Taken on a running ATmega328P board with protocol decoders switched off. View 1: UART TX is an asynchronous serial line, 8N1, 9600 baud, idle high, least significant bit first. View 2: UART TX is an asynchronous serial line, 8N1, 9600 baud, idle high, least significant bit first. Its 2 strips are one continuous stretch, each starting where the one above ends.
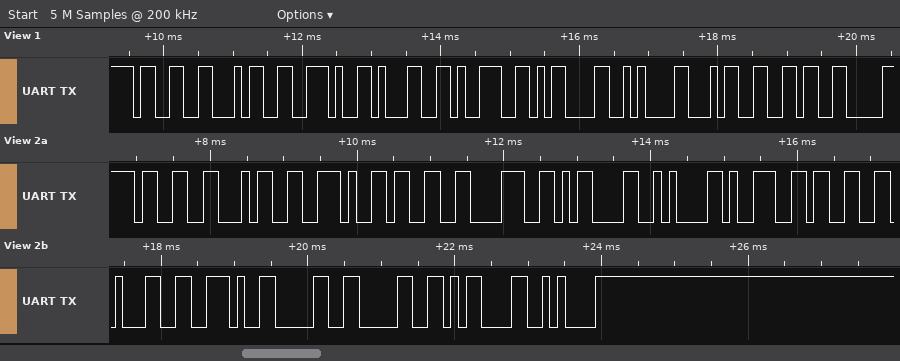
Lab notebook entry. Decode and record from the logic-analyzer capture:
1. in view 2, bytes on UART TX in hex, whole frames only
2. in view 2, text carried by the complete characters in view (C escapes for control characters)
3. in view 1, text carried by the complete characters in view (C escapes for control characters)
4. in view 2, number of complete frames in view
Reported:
33 34 2E 33 38 0D 0A 39 33 31 2E 30 30 0D 0A
"34.38\r\n931.00\r\n"
"34.19\r\n46"
15
